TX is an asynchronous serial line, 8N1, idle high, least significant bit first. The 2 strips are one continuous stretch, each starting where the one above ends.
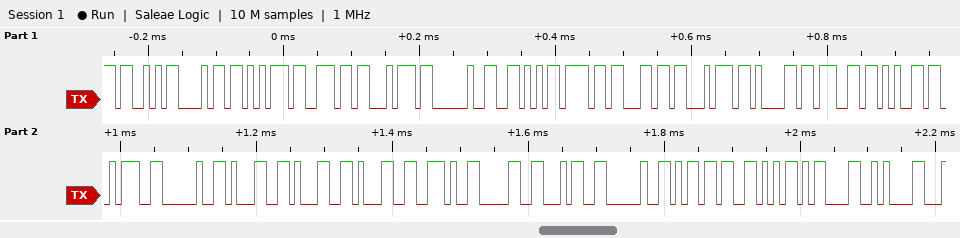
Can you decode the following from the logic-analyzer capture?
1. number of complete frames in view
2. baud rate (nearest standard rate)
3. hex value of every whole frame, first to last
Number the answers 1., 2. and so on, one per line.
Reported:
1. 26
2. 115200 baud
3. 53 68 75 6E 74 20 56 6F 6C 74 61 67 65 3A 20 31 31 31 2E 30 34 20 6D 56 0D 0A
